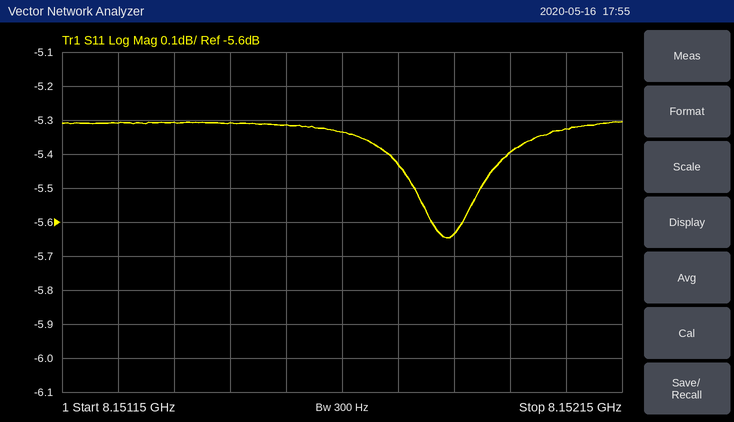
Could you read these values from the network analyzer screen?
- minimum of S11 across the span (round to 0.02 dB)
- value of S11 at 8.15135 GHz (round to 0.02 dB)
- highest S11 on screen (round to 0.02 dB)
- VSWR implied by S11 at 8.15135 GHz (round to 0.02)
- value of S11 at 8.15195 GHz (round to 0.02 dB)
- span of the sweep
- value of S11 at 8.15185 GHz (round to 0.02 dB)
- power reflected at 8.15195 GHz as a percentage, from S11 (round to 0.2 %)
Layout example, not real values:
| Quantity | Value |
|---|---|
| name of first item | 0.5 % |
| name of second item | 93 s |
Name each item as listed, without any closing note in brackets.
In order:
| Quantity | Value |
|---|---|
| minimum of S11 across the span | -5.64 dB |
| value of S11 at 8.15135 GHz | -5.30 dB |
| highest S11 on screen | -5.30 dB |
| VSWR implied by S11 at 8.15135 GHz | 3.38 |
| value of S11 at 8.15195 GHz | -5.40 dB |
| span of the sweep | 1 MHz |
| value of S11 at 8.15185 GHz | -5.64 dB |
| power reflected at 8.15195 GHz as a percentage, from S11 | 28.8 % |
